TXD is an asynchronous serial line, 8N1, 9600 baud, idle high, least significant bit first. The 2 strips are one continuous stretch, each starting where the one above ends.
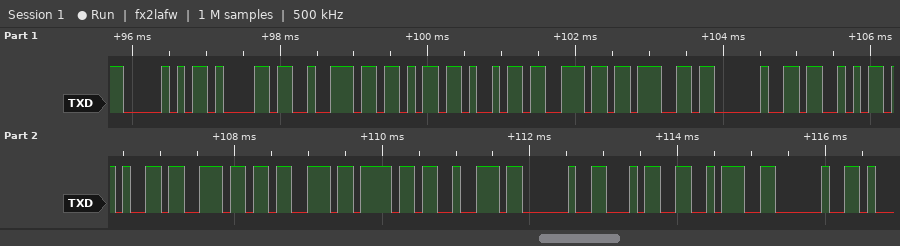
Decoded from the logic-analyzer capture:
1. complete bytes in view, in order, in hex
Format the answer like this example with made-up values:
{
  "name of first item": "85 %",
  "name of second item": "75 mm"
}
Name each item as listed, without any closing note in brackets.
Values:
{
  "complete bytes in view, in order, in hex": "0x50 0x61 0x72 0x6B 0x69 0x6E 0x67 0x20 0x53 0x65 0x6E 0x73 0x6F 0x72 0x20 0x34 0x3A 0x20"
}
